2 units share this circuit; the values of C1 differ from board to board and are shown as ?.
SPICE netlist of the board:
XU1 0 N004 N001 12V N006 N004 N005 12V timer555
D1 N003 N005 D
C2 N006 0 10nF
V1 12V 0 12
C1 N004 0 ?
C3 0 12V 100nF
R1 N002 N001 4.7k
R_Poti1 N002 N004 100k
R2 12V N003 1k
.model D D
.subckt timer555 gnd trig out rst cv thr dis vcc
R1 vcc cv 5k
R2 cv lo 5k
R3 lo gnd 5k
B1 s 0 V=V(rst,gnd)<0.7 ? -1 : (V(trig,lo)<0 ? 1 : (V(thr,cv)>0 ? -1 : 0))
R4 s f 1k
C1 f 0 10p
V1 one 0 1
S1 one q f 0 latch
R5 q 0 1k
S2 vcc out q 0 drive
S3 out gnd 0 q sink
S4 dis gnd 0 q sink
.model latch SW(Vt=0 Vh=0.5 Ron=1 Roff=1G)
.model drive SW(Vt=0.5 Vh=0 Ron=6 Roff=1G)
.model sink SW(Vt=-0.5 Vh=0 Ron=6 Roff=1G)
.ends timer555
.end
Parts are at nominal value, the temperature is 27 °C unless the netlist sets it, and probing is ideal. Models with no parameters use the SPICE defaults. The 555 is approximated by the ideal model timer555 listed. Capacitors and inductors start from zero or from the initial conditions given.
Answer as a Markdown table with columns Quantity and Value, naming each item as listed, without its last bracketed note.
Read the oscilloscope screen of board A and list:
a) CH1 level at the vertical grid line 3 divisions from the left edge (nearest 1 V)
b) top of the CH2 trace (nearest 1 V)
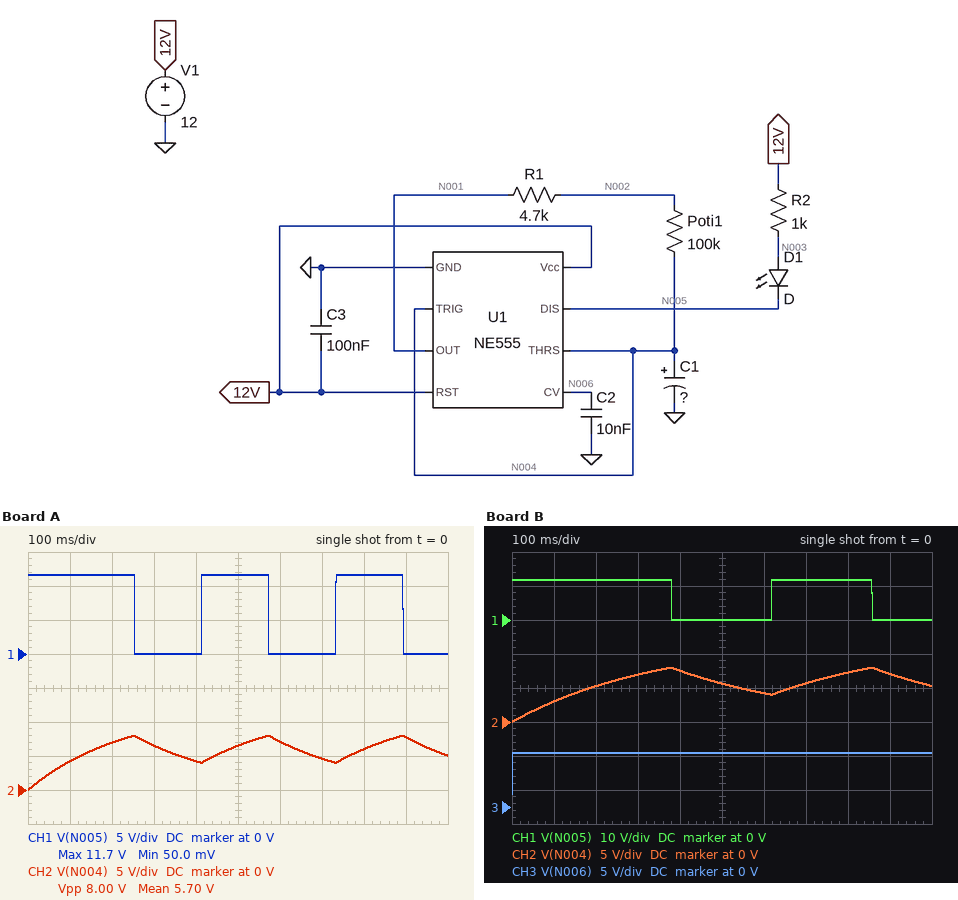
| Quantity | Value |
|---|---|
| CH1 level at the vertical grid line 3 divisions from the left edge | 0 V |
| top of the CH2 trace | 8 V |
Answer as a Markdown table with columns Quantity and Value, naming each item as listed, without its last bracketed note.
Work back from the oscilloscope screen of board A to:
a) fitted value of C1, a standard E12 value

| Quantity | Value |
|---|---|
| fitted value of C1, a standard E12 value | 2.2 µF |
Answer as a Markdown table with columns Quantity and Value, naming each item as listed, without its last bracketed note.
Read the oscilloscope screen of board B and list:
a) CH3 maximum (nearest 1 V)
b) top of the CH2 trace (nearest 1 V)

| Quantity | Value |
|---|---|
| CH3 maximum | 8 V |
| top of the CH2 trace | 8 V |
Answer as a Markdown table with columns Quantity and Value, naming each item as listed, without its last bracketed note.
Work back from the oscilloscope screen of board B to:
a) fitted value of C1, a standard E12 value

| Quantity | Value |
|---|---|
| fitted value of C1, a standard E12 value | 3.3 µF |
